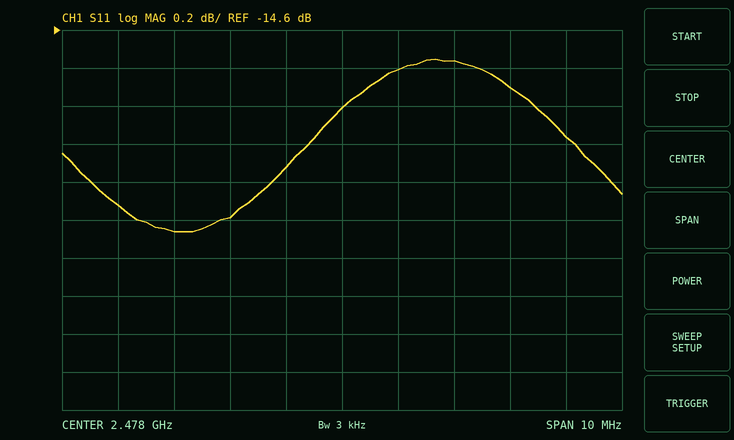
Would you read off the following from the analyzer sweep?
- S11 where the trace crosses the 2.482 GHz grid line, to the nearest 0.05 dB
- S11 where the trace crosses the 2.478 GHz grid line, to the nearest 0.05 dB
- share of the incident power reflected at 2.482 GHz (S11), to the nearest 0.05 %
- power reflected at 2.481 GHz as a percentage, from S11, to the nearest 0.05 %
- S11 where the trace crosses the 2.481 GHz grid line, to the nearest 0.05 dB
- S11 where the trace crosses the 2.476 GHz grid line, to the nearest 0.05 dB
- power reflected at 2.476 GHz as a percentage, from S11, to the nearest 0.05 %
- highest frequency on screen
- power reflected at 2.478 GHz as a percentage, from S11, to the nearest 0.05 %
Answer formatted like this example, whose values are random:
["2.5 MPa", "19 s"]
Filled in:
["-15.15 dB", "-15.00 dB", "3.05 %", "3.25 %", "-14.90 dB", "-15.60 dB", "2.75 %", "2.483 GHz", "3.15 %"]
